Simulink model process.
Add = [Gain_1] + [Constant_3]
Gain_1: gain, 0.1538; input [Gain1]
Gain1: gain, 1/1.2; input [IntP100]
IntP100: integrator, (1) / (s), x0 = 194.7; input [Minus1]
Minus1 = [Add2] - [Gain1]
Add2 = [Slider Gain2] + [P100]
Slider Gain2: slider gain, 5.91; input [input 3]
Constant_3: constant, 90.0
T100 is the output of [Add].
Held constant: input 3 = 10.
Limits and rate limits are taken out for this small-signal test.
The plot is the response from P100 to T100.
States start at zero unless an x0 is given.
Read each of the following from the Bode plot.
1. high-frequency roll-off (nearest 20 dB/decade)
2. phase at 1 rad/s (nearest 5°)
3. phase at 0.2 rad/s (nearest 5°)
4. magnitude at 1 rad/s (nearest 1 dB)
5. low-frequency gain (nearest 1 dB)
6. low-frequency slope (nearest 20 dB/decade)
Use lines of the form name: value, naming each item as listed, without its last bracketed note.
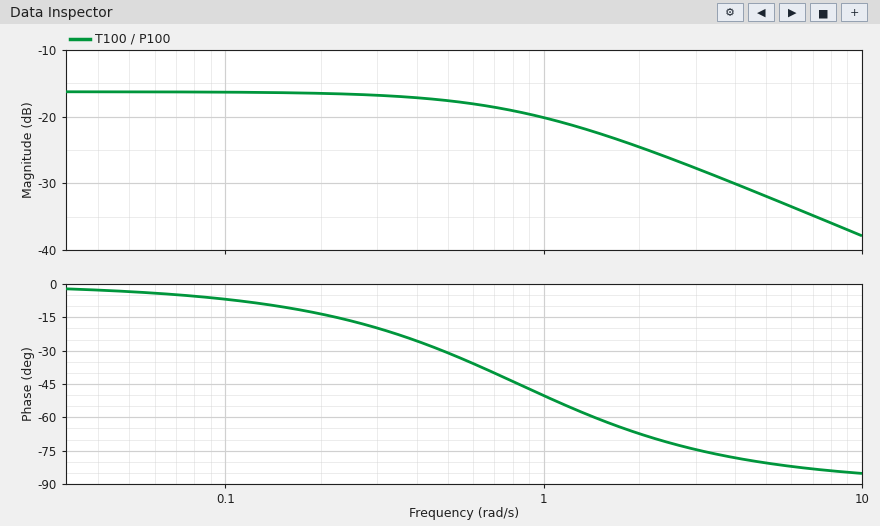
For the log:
high-frequency roll-off: -20 dB/decade
phase at 1 rad/s: -50°
phase at 0.2 rad/s: -15°
magnitude at 1 rad/s: -20 dB
low-frequency gain: -16 dB
low-frequency slope: 0 dB/decade
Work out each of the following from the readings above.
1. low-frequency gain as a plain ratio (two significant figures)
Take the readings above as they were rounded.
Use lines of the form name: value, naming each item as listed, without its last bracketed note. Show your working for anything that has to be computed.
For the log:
low-frequency gain as a plain ratio: 10^(-16 / 20) = 0.16
